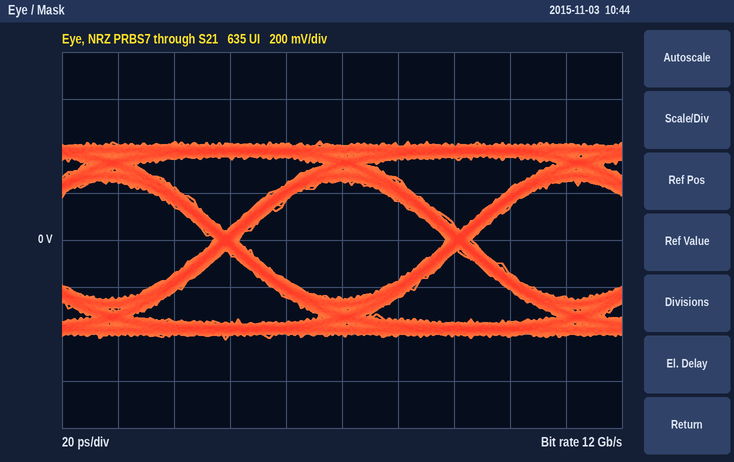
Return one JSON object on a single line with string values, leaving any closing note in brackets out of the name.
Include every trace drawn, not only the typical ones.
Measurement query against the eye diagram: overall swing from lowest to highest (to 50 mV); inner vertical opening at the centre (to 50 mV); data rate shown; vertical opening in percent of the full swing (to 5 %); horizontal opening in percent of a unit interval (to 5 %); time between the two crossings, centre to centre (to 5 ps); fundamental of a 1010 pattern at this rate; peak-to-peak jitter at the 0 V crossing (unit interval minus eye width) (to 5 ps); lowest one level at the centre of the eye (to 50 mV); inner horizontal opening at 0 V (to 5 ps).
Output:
{"overall swing from lowest to highest": "850 mV", "inner vertical opening at the centre": "500 mV", "data rate shown": "12 Gb/s", "vertical opening in percent of the full swing": "60 %", "horizontal opening in percent of a unit interval": "90 %", "time between the two crossings, centre to centre": "85 ps", "fundamental of a 1010 pattern at this rate": "6 GHz", "peak-to-peak jitter at the 0 V crossing (unit interval minus eye width)": "10 ps", "lowest one level at the centre of the eye": "250 mV", "inner horizontal opening at 0 V": "75 ps"}
